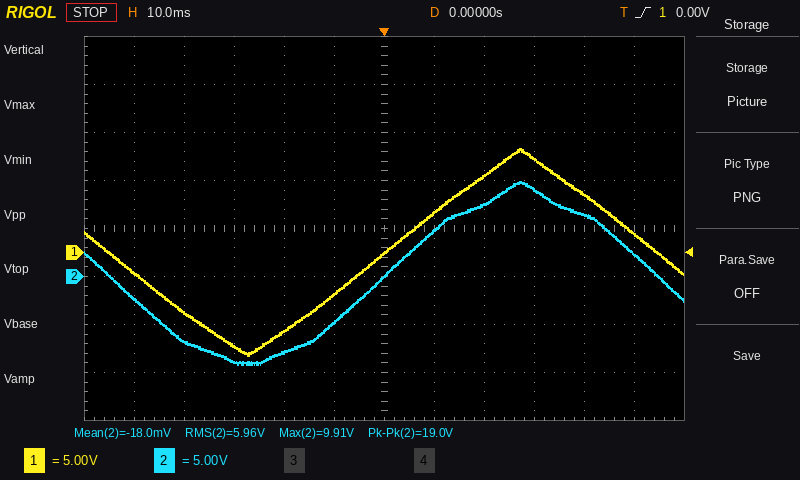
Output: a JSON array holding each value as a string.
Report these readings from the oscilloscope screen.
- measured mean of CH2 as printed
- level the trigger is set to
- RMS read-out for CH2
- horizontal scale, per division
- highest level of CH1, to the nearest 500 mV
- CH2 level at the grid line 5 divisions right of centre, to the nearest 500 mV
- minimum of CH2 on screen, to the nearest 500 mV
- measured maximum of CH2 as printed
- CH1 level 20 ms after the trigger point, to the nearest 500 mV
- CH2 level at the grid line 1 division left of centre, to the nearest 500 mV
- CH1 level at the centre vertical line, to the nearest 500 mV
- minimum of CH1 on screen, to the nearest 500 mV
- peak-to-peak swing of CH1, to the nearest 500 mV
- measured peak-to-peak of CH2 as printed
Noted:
["-18.0 mV", "0.00 V", "5.96 V", "10 ms", "11.0 V", "2.5 V", "-9.0 V", "9.91 V", "8.0 V", "-5.0 V", "0.0 V", "-10.5 V", "21.5 V", "19.0 V"]
